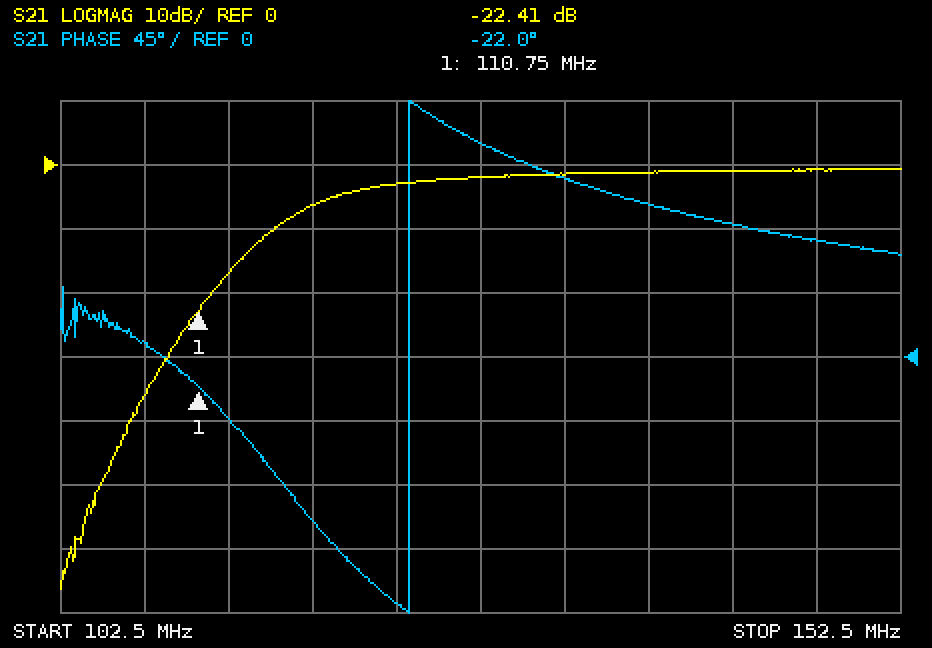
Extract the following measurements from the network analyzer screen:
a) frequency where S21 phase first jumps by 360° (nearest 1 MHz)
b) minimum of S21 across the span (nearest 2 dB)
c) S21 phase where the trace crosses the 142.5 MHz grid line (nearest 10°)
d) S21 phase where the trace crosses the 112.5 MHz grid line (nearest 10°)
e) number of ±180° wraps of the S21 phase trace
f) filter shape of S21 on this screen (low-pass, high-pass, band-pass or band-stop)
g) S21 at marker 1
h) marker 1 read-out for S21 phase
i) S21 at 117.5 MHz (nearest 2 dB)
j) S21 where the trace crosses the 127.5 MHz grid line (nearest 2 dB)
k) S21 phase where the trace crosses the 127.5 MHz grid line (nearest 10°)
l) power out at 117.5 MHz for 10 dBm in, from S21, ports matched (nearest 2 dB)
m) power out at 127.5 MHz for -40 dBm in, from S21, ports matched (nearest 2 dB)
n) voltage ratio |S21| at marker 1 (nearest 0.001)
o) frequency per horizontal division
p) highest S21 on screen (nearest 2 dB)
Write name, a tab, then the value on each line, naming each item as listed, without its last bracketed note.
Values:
frequency where S21 phase first jumps by 360°	123 MHz
minimum of S21 across the span	-66 dB
S21 phase where the trace crosses the 142.5 MHz grid line	90°
S21 phase where the trace crosses the 112.5 MHz grid line	-40°
number of ±180° wraps of the S21 phase trace	1
filter shape of S21 on this screen	high-pass
S21 at marker 1	-22.41 dB
marker 1 read-out for S21 phase	-22.0°
S21 at 117.5 MHz	-6 dB
S21 where the trace crosses the 127.5 MHz grid line	-2 dB
S21 phase where the trace crosses the 127.5 MHz grid line	150°
power out at 117.5 MHz for 10 dBm in, from S21, ports matched	4 dBm
power out at 127.5 MHz for -40 dBm in, from S21, ports matched	-42 dBm
voltage ratio |S21| at marker 1	0.076
frequency per horizontal division	5 MHz
highest S21 on screen	0 dB
